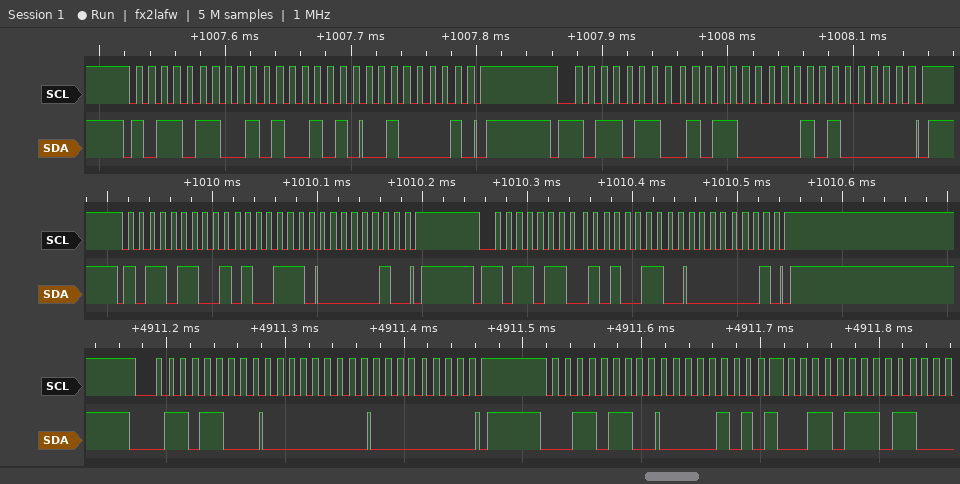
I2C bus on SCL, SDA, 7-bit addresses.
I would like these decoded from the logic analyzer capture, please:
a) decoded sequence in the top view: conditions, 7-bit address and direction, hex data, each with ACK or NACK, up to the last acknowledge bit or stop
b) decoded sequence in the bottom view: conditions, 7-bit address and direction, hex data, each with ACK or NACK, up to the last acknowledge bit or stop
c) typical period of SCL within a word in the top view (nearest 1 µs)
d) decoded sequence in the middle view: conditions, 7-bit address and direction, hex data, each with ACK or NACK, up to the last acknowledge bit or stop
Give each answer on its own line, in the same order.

start, address 5B write ACK, A5 ACK, 21 ACK, stop, start, address 5B write ACK, B0 ACK, A0 ACK, stop
start, address 36 write ACK, 00 ACK, 00 ACK, stop, start, address 1B write ACK, 05 ACK, repeated start, address 1B read ACK
10 µs
start, address 5B write ACK, A7 ACK, 02 ACK, stop, start, address 5B write ACK, A6 ACK, 01 ACK, stop
